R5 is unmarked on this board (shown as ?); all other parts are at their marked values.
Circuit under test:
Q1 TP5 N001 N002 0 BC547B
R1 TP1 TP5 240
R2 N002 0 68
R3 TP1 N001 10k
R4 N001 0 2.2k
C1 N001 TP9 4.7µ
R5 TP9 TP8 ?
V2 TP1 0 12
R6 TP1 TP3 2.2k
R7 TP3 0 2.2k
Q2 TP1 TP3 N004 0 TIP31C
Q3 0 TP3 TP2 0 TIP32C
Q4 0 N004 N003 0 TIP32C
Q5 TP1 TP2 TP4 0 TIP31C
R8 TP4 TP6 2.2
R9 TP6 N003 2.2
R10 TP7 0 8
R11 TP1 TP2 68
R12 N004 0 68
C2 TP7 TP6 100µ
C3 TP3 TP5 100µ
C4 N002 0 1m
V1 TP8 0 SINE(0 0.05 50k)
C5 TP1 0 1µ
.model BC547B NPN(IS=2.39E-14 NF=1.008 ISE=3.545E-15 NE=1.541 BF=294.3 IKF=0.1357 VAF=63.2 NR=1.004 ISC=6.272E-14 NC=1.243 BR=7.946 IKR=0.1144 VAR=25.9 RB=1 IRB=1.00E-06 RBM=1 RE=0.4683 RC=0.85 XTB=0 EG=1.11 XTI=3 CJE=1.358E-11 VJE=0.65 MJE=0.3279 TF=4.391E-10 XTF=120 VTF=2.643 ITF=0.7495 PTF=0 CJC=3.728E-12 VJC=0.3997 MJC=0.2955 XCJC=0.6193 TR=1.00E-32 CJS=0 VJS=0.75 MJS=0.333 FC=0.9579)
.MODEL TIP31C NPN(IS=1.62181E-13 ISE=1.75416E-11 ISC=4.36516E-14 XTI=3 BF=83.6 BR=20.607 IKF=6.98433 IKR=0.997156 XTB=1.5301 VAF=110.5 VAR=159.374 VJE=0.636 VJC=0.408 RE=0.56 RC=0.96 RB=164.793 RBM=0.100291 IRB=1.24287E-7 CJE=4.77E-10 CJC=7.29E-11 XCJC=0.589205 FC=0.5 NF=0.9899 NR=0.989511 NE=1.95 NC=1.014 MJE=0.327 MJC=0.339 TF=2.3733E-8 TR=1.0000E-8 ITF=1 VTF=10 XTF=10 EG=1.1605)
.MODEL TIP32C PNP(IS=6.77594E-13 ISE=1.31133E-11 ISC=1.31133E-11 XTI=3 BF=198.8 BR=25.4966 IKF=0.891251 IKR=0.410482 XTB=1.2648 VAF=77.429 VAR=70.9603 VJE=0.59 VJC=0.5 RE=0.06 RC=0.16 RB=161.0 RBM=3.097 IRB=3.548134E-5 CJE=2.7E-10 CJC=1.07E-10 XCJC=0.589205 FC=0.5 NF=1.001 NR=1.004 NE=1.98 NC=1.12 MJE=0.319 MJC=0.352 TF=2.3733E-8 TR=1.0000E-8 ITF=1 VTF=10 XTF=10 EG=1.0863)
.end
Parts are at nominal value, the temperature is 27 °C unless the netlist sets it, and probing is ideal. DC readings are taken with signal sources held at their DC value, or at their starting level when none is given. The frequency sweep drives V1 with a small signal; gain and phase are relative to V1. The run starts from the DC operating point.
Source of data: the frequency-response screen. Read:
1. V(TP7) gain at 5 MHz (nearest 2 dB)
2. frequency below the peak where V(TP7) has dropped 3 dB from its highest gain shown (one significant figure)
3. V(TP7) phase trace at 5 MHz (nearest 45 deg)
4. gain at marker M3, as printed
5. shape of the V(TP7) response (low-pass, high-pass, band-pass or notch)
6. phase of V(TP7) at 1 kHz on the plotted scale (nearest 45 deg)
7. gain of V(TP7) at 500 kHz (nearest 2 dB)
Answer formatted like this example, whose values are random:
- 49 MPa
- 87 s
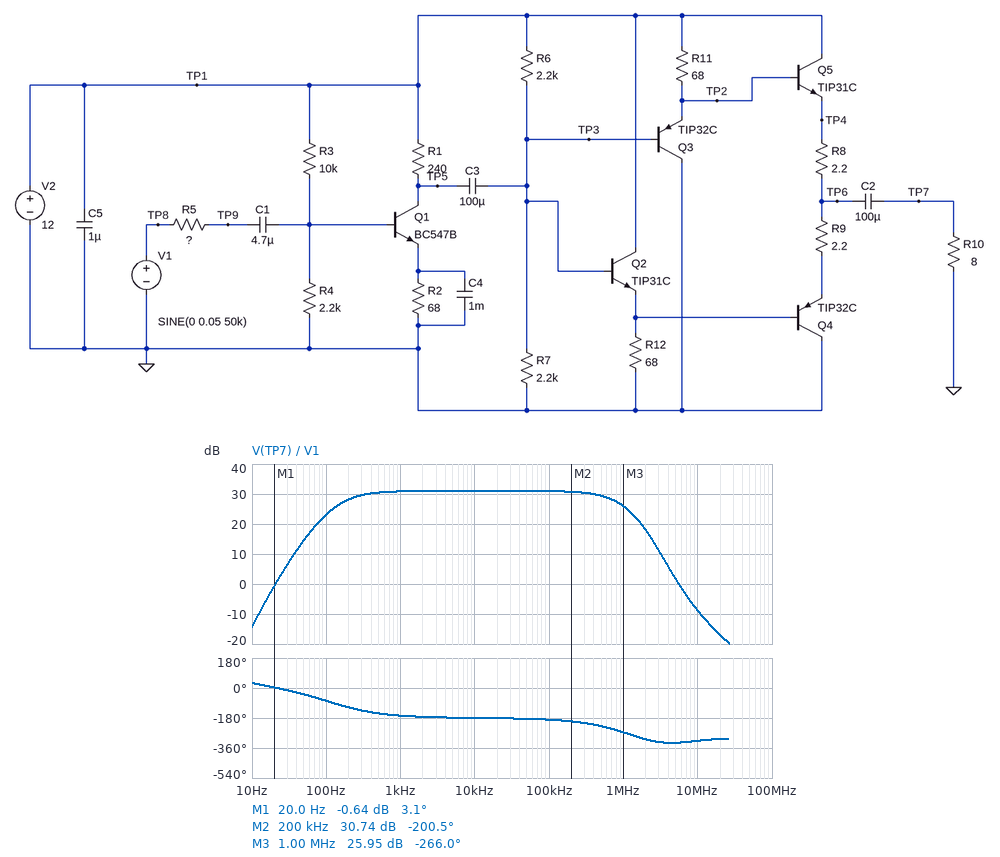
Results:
- 2 dB
- 200 Hz
- -315 deg
- 25.95 dB
- band-pass
- -180 deg
- 30 dB
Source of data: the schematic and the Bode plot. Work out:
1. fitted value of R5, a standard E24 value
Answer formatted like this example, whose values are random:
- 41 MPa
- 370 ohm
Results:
- 390 Ω
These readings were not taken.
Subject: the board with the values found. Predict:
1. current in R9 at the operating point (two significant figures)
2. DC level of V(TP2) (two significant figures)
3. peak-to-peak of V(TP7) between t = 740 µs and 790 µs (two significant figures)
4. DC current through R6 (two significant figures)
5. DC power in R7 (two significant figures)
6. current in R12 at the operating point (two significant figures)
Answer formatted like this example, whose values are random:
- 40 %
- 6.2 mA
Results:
- 23 mA
- 6.3 V
- 3.2 V
- 2.9 mA
- 14 mW
- 71 mA
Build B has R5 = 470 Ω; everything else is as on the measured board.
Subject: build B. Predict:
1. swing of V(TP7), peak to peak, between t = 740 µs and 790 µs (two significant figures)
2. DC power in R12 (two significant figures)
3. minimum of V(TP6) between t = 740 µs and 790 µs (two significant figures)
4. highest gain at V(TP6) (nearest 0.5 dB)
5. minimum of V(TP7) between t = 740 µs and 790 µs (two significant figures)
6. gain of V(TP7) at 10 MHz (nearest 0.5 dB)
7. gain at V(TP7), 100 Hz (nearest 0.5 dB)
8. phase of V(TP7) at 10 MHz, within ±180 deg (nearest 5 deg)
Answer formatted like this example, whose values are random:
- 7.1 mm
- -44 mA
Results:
- 2.9 V
- 350 mW
- 4.0 V
- 30.5 dB
- -1.5 V
- -10.5 dB
- 22.5 dB
- 40 deg
